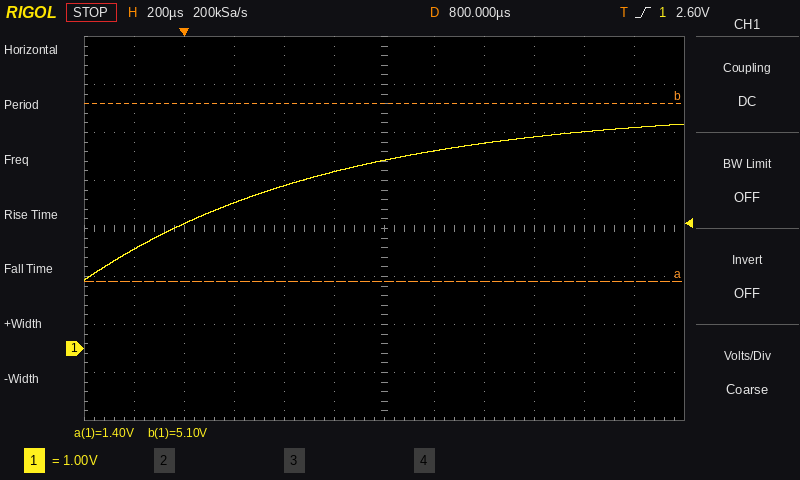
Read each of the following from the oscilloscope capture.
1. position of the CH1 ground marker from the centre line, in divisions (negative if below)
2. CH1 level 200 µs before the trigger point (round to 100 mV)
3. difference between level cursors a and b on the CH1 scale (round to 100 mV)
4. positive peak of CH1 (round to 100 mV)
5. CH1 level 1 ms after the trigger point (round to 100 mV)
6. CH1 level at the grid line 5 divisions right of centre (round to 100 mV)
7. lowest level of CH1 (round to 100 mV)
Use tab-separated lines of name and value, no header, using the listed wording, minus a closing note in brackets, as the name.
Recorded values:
position of the CH1 ground marker from the centre line, in divisions	-2.5 div
CH1 level 200 µs before the trigger point	2.1 V
difference between level cursors a and b on the CH1 scale	3.7 V
positive peak of CH1	4.7 V
CH1 level 1 ms after the trigger point	4.1 V
CH1 level at the grid line 5 divisions right of centre	4.6 V
lowest level of CH1	1.4 V
